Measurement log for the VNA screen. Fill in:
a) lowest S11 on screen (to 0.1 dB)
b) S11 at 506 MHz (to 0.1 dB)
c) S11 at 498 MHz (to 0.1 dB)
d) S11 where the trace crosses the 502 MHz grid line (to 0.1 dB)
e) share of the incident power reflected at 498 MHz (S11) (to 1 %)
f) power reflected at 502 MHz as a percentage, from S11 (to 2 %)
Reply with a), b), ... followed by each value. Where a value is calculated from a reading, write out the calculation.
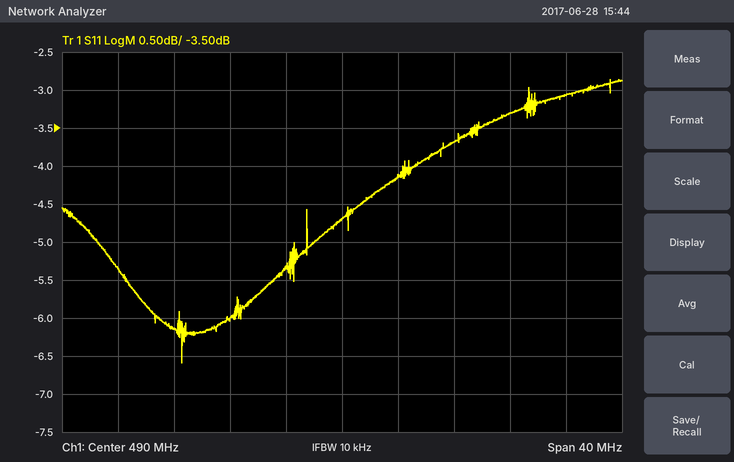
a) -6.6 dB
b) -3.1 dB
c) -3.7 dB
d) -3.3 dB
e) 10^(-3.7/10) ≈ 43 %
f) 10^(-3.3/10) ≈ 46.8 %, so 46 % to the nearest 2 %
